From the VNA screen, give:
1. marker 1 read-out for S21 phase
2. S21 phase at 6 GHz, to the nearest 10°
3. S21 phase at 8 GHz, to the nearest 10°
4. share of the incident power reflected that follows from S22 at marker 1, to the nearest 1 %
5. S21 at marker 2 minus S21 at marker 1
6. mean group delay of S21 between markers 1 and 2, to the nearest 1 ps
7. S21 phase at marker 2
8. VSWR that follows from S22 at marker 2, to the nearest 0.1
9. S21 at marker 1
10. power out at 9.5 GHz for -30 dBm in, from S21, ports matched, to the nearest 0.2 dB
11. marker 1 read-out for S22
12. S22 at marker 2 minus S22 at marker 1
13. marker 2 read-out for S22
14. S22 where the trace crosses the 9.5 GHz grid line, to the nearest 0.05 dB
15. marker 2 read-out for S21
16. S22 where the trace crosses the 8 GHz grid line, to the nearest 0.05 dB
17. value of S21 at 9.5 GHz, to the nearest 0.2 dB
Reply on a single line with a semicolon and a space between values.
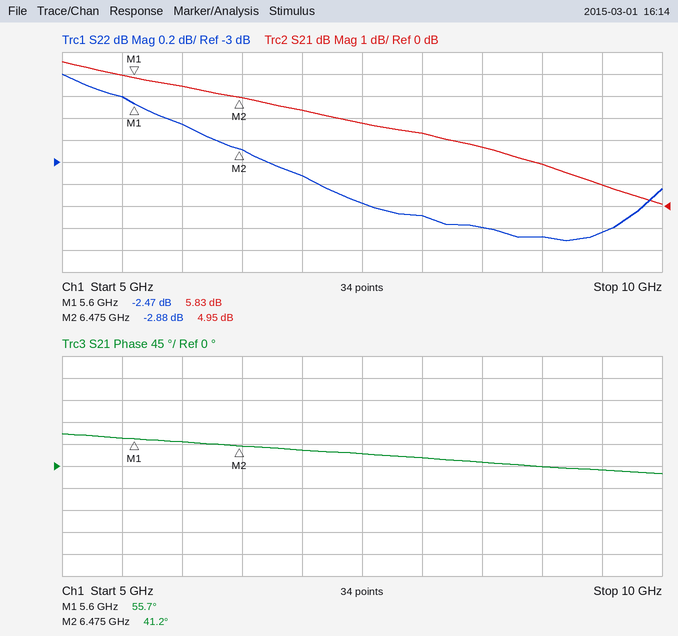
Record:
55.7°; 50°; 20°; 57 %; -0.88 dB; 46 ps; 41.2°; 6.1; 5.83 dB; -29.0 dBm; -2.47 dB; -0.41 dB; -2.88 dB; -3.65 dB; 4.95 dB; -3.50 dB; 1.0 dB
